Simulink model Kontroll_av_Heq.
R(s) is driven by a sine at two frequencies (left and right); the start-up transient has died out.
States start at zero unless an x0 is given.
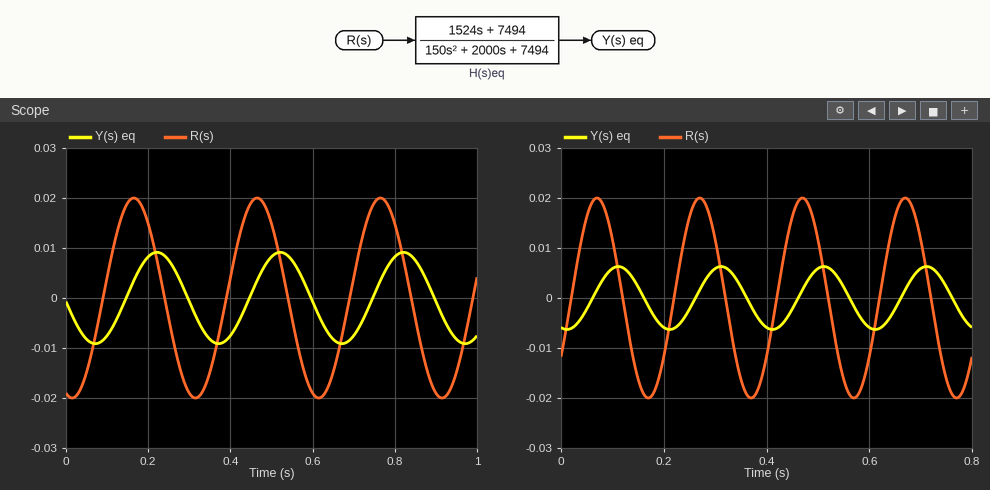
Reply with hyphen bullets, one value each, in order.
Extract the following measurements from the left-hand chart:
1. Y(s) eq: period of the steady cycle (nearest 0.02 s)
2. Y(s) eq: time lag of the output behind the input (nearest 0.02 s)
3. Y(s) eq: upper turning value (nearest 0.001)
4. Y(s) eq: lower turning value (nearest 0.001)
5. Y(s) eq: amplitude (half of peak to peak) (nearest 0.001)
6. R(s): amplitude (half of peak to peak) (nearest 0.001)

- 0.30 s
- 0.06 s
- 0.009
- -0.009
- 0.009
- 0.020
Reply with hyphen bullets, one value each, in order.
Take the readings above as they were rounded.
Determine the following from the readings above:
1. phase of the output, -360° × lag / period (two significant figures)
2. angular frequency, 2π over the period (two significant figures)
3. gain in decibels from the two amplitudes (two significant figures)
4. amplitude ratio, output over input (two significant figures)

- -72°
- 21 rad/s
- -6.9 dB
- 0.45
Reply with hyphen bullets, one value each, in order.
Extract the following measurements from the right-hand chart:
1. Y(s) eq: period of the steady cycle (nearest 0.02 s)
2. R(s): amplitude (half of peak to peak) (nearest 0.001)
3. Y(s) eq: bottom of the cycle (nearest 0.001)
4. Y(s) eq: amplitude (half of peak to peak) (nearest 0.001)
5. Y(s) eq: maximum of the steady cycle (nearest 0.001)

- 0.20 s
- 0.020
- -0.006
- 0.006
- 0.006
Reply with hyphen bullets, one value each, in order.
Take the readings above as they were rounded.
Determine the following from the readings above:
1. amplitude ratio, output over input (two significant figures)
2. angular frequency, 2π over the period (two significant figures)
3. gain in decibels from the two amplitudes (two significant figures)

- 0.30
- 31 rad/s
- -10 dB
